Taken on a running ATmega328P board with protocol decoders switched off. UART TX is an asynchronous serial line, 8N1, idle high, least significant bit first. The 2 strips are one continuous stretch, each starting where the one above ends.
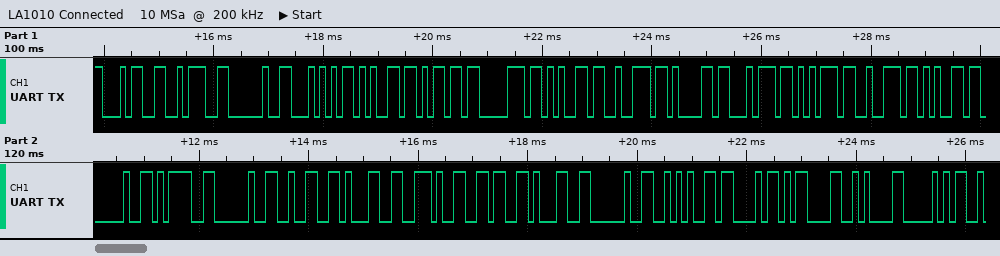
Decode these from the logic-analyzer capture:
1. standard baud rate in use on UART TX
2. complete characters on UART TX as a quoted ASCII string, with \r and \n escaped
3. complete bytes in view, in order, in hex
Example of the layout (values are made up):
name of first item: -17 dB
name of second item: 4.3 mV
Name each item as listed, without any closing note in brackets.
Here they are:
standard baud rate in use on UART TX: 9600 baud
complete characters on UART TX as a quoted ASCII string, with \r and \n escaped: "4: Temperature = 21.61 *C\r\nP"
complete bytes in view, in order, in hex: 34 3A 20 54 65 6D 70 65 72 61 74 75 72 65 20 3D 20 32 31 2E 36 31 20 2A 43 0D 0A 50
